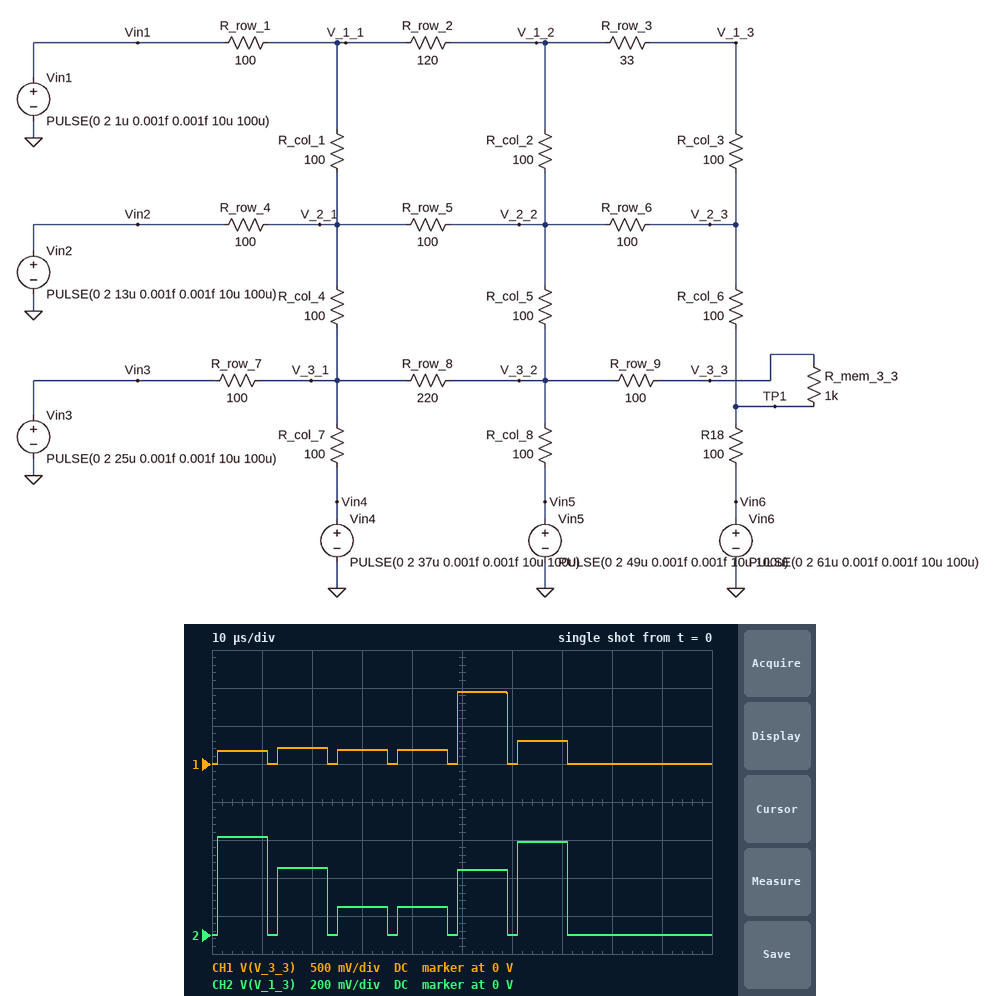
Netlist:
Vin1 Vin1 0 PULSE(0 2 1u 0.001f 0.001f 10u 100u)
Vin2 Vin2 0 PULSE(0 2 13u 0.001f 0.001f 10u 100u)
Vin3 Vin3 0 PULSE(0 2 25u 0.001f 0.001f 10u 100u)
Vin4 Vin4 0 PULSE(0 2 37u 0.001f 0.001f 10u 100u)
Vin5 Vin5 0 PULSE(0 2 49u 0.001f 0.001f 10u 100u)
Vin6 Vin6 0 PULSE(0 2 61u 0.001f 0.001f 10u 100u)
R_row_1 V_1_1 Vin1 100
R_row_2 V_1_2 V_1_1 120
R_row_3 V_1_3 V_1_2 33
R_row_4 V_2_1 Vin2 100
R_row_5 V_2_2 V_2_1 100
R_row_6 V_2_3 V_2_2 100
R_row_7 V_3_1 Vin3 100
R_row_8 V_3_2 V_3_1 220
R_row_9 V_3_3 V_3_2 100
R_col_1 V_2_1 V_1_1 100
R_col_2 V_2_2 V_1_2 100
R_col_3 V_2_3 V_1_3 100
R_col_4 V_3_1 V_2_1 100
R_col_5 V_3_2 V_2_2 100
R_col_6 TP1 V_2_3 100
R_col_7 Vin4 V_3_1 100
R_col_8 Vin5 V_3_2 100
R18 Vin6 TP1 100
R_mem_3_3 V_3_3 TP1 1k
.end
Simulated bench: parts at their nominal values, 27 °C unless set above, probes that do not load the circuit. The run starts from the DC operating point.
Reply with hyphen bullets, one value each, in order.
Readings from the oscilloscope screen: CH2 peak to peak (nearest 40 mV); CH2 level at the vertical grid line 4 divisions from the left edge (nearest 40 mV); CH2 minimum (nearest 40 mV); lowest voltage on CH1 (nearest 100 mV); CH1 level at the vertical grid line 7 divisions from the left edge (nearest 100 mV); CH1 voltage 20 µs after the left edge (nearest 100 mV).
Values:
- 520 mV
- 160 mV
- 0 V
- 0 V
- 300 mV
- 200 mV
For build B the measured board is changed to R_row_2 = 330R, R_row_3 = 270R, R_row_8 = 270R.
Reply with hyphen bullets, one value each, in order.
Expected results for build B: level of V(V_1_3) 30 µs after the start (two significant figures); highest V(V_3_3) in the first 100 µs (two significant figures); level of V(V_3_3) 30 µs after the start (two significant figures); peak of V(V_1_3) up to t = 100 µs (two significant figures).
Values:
- 140 mV
- 980 mV
- 170 mV
- 720 mV
